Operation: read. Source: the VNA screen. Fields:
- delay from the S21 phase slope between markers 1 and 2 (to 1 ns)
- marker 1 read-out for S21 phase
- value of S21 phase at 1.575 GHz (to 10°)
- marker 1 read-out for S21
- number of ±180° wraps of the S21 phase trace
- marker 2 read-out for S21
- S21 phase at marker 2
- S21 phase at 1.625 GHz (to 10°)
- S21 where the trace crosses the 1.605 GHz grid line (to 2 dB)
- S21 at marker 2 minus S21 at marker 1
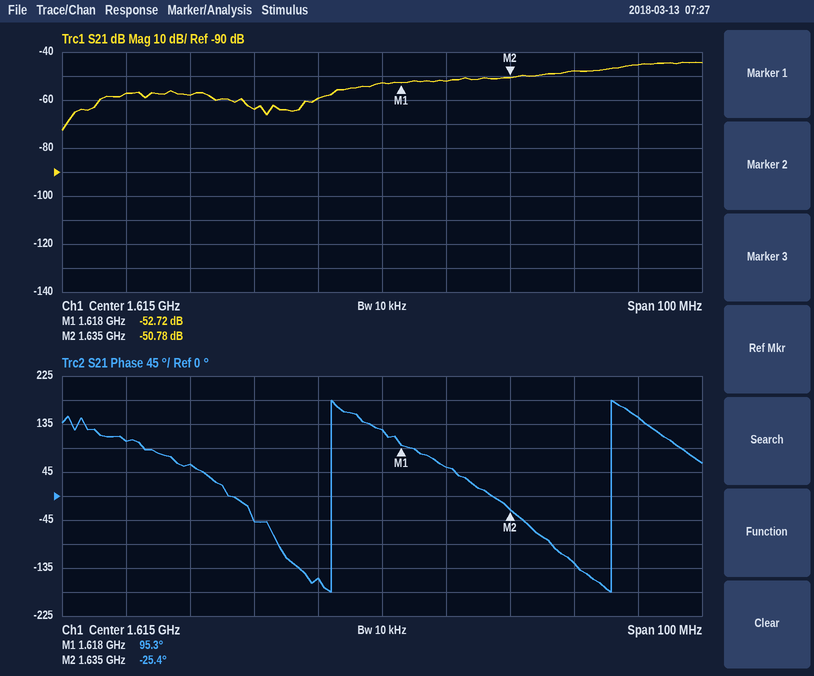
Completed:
20 ns
95.3°
100°
-52.72 dB
2
-50.78 dB
-25.4°
50°
-60 dB
1.94 dB
